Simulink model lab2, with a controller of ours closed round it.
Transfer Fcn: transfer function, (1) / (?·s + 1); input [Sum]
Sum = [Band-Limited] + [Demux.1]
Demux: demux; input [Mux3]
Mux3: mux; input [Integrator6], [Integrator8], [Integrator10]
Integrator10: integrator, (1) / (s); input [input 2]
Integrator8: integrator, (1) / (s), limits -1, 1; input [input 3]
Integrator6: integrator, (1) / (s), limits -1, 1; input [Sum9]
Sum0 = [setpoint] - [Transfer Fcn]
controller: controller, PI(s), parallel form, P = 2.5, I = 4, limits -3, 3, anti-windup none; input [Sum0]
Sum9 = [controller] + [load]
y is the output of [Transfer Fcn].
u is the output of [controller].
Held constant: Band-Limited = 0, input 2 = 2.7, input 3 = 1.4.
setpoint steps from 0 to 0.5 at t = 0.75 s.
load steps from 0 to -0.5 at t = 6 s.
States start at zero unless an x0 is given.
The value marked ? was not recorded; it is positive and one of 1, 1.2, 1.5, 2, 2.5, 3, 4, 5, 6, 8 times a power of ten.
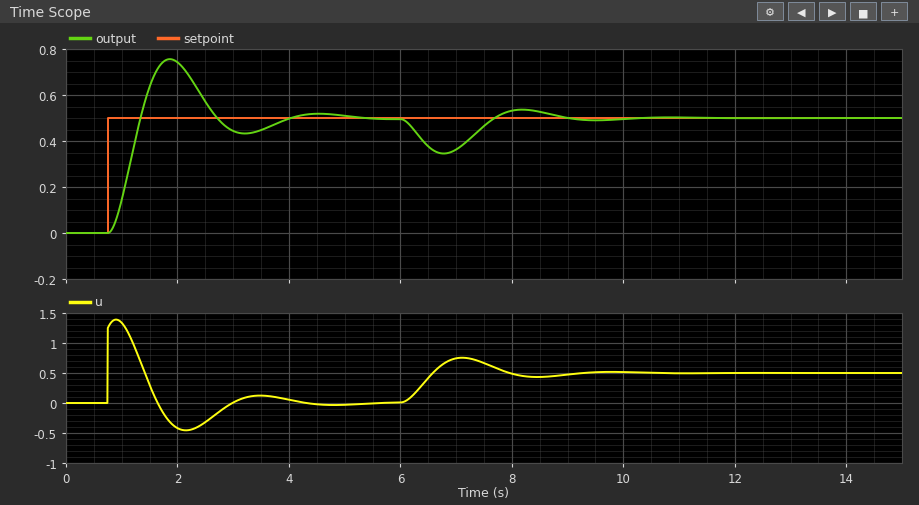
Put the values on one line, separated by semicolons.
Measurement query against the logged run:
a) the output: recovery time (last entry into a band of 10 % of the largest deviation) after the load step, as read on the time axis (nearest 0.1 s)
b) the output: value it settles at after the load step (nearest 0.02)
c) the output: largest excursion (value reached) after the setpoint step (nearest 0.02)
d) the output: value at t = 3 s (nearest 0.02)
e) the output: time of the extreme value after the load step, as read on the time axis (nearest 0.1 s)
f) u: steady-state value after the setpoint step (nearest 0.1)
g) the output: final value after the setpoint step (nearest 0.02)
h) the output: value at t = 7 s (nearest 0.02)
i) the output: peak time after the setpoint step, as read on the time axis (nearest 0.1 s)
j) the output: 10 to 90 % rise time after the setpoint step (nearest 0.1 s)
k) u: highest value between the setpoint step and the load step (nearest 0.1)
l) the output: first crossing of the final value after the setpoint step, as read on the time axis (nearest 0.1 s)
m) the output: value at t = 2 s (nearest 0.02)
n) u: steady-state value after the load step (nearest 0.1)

8.7 s; 0.50; 0.76; 0.44; 6.8 s; 0.0; 0.50; 0.36; 1.9 s; 0.4 s; 1.4; 1.3 s; 0.74; 0.5
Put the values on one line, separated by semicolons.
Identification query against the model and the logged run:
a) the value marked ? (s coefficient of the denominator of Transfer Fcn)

0.2
